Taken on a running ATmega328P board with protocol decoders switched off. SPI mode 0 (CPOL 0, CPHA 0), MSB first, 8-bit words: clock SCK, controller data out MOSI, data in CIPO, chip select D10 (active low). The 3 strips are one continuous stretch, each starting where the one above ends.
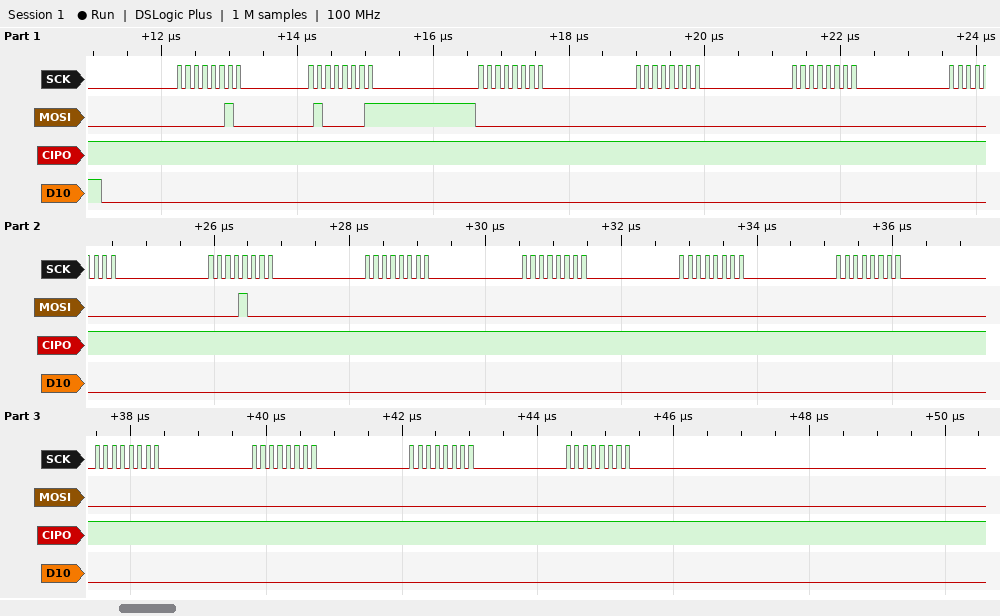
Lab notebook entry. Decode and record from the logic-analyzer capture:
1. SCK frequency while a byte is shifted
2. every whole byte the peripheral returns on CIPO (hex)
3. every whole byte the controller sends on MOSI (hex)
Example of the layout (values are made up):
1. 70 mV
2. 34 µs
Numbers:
1. 8 MHz
2. FF FF FF FF FF FF FF FF FF FF FF FF FF FF FF
3. 02 41 00 00 00 00 08 00 00 00 00 00 00 00 00
